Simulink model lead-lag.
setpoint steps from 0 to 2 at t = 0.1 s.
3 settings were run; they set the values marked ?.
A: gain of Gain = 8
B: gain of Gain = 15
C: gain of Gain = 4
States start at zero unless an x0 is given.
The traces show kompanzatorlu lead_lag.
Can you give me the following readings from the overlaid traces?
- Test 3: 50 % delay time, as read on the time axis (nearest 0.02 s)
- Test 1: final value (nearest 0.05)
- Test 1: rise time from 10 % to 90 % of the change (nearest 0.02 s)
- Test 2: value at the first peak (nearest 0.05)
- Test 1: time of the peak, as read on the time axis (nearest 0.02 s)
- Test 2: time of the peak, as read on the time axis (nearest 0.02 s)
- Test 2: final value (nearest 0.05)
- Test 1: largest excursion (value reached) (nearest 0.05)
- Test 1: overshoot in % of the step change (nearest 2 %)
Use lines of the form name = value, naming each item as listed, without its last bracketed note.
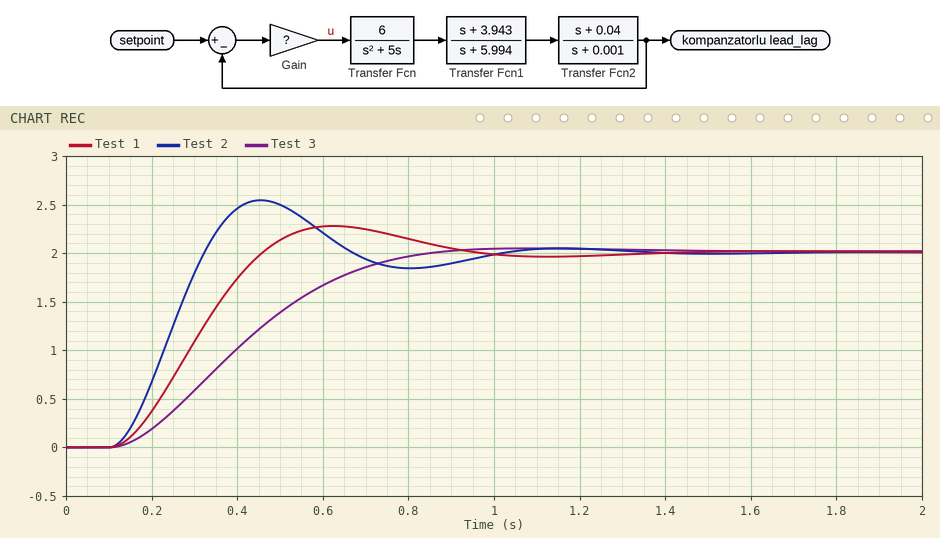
Test 3: 50 % delay time, as read on the time axis = 0.40 s
Test 1: final value = 2.00
Test 1: rise time from 10 % to 90 % of the change = 0.24 s
Test 2: value at the first peak = 2.55
Test 1: time of the peak, as read on the time axis = 0.62 s
Test 2: time of the peak, as read on the time axis = 0.46 s
Test 2: final value = 2.00
Test 1: largest excursion (value reached) = 2.30
Test 1: overshoot in % of the step change = 14 %
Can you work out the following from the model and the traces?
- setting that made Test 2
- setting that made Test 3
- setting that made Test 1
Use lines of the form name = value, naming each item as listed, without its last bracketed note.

setting that made Test 2 = B
setting that made Test 3 = C
setting that made Test 1 = A
